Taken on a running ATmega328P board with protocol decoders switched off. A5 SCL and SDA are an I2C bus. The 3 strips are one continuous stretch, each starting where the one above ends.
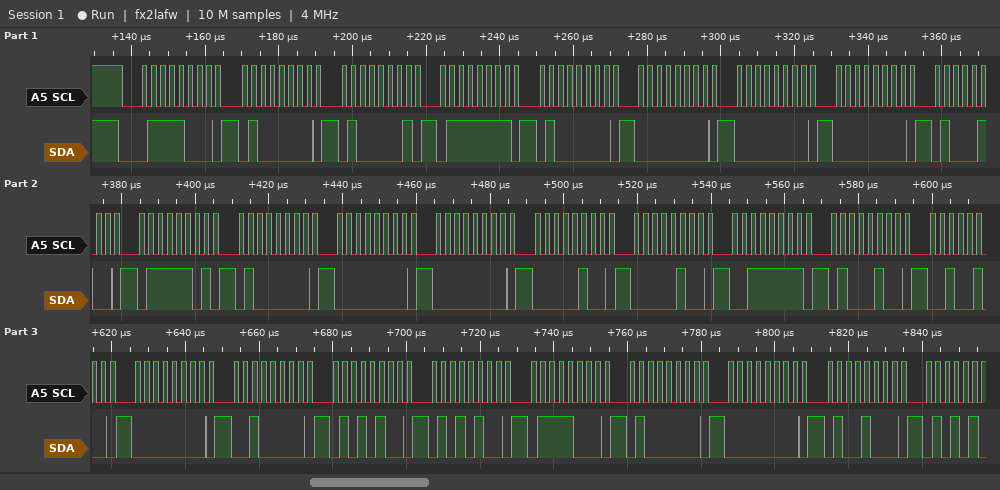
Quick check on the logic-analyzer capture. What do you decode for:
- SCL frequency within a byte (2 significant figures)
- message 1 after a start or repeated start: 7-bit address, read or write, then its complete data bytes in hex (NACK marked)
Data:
400 kHz
0x3C write: 40 41 7F 40 00 00 00 44 7D 40 00 00 04 04 3F 44 24 00 20 54 54 78 40 00 48
